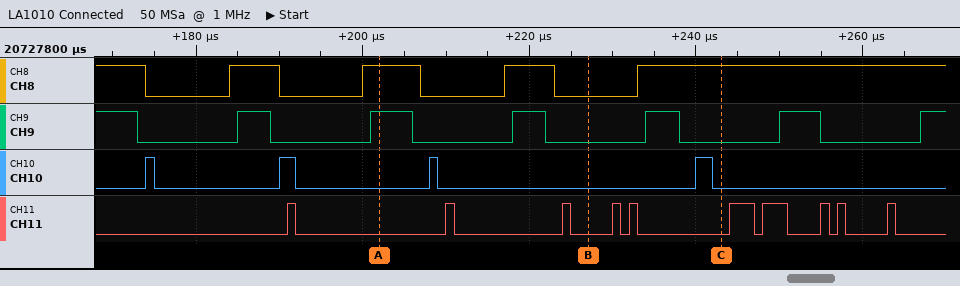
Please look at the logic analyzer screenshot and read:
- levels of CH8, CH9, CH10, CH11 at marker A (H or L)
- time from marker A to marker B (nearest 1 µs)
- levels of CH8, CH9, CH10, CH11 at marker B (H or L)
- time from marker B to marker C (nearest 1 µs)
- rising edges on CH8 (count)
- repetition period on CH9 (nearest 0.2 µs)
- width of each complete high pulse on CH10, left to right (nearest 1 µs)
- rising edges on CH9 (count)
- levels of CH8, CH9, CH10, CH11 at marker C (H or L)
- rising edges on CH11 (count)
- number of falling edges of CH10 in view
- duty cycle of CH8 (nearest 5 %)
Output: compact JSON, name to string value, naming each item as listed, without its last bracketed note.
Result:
{"levels of CH8, CH9, CH10, CH11 at marker A": "CH8=H, CH9=H, CH10=L, CH11=L", "time from marker A to marker B": "25 µs", "levels of CH8, CH9, CH10, CH11 at marker B": "CH8=L, CH9=L, CH10=L, CH11=L", "time from marker B to marker C": "16 µs", "rising edges on CH8": "4", "repetition period on CH9": "16.4 µs", "width of each complete high pulse on CH10, left to right": "1 µs, 2 µs, 1 µs, 2 µs", "rising edges on CH9": "6", "levels of CH8, CH9, CH10, CH11 at marker C": "CH8=H, CH9=L, CH10=L, CH11=L", "rising edges on CH11": "10", "number of falling edges of CH10 in view": "4", "duty cycle of CH8": "40 %"}
